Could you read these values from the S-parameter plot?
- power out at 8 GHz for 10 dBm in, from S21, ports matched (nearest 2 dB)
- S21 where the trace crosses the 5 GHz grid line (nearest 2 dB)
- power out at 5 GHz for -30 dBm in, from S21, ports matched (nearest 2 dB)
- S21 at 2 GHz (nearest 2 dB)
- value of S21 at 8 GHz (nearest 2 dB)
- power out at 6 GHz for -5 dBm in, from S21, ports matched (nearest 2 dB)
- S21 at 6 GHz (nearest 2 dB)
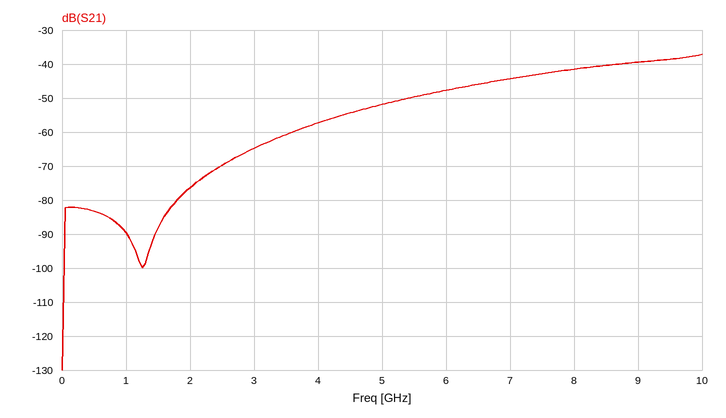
-32 dBm
-52 dB
-82 dBm
-76 dB
-42 dB
-52 dBm
-48 dB
